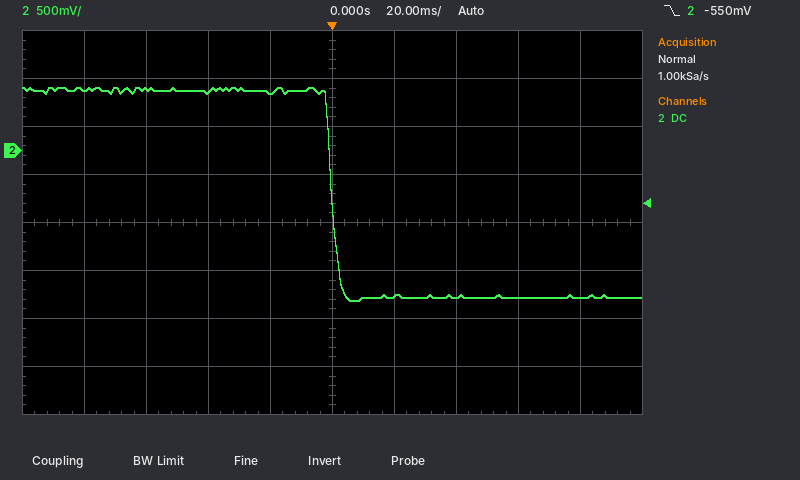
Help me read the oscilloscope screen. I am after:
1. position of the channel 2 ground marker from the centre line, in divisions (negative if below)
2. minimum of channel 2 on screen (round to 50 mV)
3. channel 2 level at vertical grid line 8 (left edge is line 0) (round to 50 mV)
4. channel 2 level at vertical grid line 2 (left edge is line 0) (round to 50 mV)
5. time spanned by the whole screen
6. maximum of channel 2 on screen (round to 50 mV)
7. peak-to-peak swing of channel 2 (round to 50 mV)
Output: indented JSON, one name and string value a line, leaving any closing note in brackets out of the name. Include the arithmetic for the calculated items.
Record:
{
  "position of the channel 2 ground marker from the centre line, in divisions": "+1.5 div",
  "minimum of channel 2 on screen": "-1.55 V",
  "channel 2 level at vertical grid line 8 (left edge is line 0)": "-1.55 V",
  "channel 2 level at vertical grid line 2 (left edge is line 0)": "650 mV",
  "time spanned by the whole screen": "200 ms",
  "maximum of channel 2 on screen": "650 mV",
  "peak-to-peak swing of channel 2": "650 mV − (-1.55 V) = 2.20 V"
}
